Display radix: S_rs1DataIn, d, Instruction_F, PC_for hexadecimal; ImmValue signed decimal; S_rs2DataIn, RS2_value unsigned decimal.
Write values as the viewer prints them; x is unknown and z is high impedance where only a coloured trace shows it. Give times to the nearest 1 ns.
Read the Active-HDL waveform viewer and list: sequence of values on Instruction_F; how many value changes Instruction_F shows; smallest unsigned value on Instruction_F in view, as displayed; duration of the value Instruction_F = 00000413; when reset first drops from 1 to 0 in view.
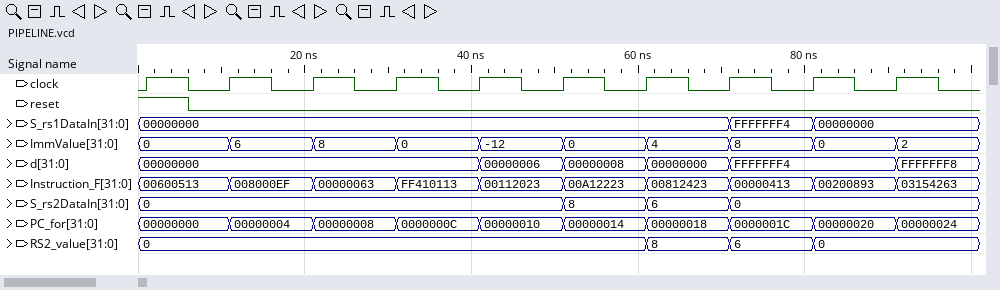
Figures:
00600513, 008000EF, 00000063, FF410113, 00112023, 00A12223, 00812423, 00000413, 00200893, 03154263
9
00000063
10 ns
6 ns
